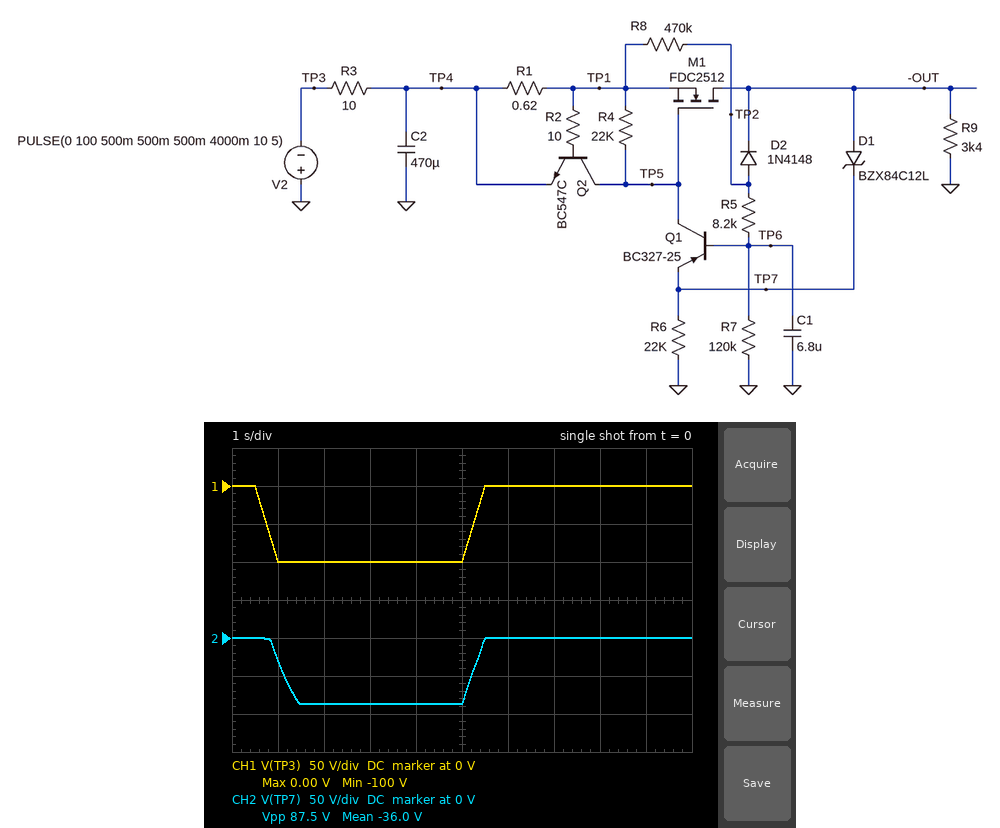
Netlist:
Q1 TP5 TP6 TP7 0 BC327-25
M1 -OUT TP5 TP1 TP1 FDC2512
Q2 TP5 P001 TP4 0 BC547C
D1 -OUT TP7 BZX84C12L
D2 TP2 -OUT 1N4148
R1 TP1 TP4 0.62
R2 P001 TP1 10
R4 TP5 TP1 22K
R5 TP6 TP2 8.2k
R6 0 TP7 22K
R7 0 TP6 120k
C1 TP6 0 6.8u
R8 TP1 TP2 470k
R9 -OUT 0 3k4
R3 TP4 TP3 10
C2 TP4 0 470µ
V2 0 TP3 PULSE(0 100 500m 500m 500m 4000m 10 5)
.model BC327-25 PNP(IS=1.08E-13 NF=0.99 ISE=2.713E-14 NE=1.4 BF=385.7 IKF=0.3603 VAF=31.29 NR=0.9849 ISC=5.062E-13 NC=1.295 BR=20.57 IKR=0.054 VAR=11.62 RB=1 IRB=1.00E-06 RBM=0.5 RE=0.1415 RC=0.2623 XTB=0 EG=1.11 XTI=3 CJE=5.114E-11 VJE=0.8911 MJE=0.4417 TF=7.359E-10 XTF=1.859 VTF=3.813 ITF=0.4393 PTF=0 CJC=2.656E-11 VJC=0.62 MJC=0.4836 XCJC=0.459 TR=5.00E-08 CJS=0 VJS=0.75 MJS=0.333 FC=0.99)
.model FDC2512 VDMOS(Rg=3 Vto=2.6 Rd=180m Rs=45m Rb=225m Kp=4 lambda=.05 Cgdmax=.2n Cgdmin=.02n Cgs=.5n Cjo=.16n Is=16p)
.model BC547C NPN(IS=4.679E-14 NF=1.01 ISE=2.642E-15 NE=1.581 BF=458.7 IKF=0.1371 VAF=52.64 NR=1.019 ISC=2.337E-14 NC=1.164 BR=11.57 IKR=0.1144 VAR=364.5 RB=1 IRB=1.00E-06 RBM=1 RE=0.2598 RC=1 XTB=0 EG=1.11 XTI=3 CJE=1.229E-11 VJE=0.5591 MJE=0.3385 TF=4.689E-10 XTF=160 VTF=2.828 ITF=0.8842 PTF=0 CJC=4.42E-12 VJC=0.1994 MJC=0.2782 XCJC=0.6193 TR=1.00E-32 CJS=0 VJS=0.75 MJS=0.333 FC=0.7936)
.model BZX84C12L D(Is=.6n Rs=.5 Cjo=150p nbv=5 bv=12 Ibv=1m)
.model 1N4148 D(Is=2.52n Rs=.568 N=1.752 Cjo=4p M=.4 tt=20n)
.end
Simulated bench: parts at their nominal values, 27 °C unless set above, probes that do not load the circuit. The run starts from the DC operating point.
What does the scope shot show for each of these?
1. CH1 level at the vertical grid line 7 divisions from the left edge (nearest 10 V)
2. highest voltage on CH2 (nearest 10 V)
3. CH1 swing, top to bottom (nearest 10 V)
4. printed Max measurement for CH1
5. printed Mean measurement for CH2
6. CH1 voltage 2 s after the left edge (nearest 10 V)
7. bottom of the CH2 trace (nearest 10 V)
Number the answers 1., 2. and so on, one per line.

1. 0 V
2. 0 V
3. 100 V
4. 0.00 V
5. -36.0 V
6. -100 V
7. -90 V
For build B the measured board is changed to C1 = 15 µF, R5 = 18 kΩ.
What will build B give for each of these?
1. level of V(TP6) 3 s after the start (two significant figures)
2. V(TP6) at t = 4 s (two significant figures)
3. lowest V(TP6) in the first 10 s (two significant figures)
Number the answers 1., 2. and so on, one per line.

1. -50 V
2. -60 V
3. -66 V
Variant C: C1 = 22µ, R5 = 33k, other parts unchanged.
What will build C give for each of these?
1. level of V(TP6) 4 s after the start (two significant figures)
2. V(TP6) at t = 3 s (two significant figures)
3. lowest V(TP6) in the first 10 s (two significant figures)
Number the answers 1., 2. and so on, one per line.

1. -27 V
2. -22 V
3. -32 V
